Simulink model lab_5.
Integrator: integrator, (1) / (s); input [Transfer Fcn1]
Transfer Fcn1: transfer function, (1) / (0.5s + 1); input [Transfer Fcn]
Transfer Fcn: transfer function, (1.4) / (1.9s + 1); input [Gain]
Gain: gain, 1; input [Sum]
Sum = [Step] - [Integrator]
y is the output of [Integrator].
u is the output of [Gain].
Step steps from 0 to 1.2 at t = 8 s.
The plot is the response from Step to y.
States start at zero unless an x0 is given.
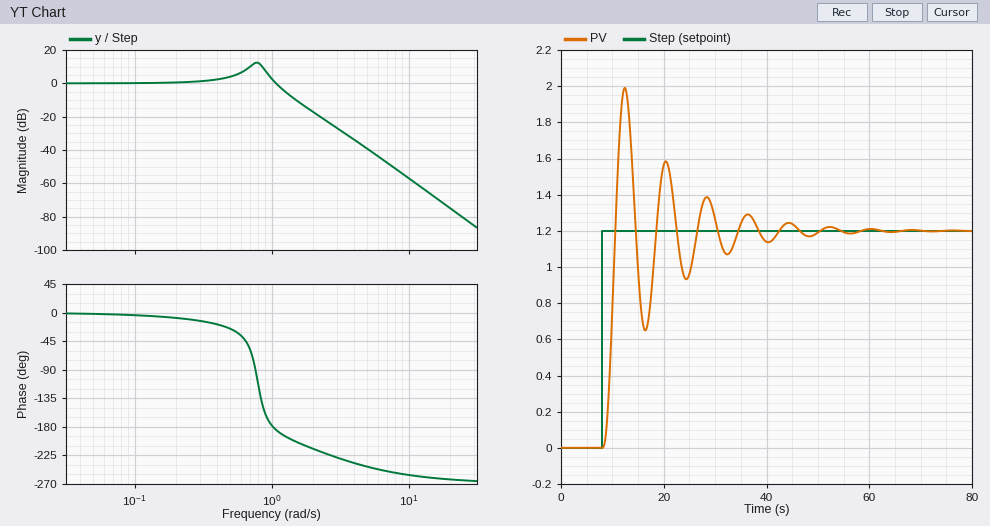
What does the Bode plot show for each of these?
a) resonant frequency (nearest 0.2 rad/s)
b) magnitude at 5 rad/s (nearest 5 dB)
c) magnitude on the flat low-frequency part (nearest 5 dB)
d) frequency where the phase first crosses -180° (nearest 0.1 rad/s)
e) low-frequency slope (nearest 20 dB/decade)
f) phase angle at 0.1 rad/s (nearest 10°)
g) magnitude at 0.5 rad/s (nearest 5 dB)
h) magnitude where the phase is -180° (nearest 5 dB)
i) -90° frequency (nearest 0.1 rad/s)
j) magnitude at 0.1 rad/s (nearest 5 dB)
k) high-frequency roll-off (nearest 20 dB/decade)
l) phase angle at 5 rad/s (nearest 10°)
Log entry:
0.8 rad/s
-40 dB
0 dB
1.0 rad/s
0 dB/decade
0°
5 dB
0 dB
0.8 rad/s
0 dB
-60 dB/decade
-240°
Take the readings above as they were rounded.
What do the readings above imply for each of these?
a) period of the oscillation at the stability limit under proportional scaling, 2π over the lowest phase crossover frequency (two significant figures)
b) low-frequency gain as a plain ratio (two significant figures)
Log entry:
6.3 s
1.0
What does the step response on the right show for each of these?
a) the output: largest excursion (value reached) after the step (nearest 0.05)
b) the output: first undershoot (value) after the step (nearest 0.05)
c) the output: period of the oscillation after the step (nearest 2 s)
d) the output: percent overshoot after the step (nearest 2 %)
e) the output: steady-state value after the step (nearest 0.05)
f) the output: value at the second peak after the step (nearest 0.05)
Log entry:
2.00
0.65
8 s
66 %
1.20
1.60
